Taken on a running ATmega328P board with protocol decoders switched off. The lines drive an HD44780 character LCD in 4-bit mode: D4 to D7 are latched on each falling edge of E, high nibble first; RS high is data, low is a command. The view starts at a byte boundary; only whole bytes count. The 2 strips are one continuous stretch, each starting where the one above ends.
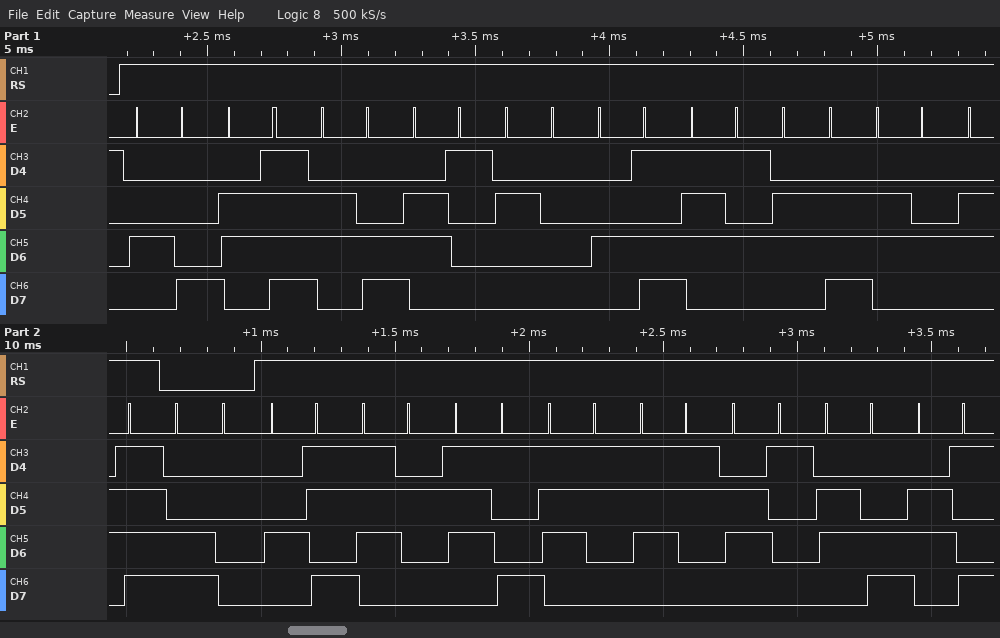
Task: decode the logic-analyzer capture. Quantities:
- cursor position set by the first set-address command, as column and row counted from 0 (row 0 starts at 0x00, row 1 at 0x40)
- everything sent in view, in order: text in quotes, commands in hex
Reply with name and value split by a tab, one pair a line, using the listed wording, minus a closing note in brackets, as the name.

cursor position set by the first set-address command, as column and row counted from 0	column 0, row 1
everything sent in view, in order: text in quotes, commands in hex	"Hola Mundo" 0xC0 "Kryssali"
